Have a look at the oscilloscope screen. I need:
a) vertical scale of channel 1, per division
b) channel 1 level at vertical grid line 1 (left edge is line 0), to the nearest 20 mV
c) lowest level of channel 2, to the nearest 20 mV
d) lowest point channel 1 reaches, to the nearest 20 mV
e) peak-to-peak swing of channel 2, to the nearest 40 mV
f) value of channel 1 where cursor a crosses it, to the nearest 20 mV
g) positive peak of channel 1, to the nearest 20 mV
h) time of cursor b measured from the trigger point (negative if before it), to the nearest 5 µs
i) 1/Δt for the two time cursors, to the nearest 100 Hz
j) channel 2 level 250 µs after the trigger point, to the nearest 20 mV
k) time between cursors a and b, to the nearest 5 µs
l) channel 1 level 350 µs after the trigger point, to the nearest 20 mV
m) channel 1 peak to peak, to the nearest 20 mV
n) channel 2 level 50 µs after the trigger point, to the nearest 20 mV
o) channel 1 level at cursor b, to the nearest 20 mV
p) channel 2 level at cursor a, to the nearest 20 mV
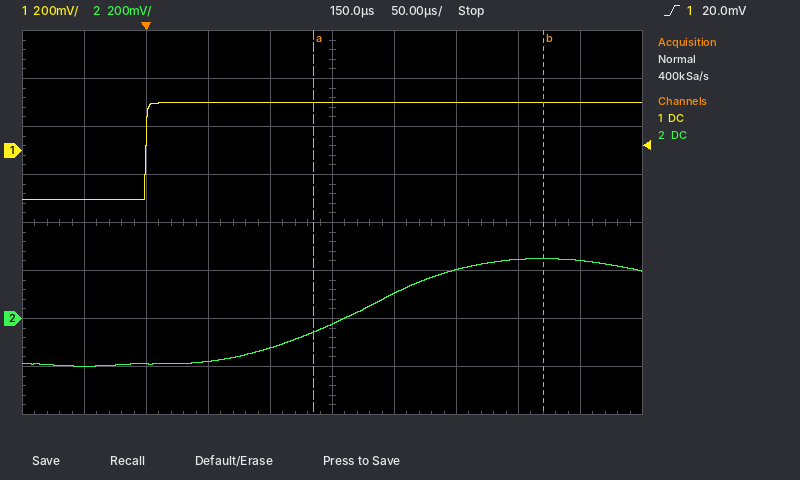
200 mV
-200 mV
-200 mV
-200 mV
440 mV
200 mV
200 mV
+320 µs
5.4 kHz
200 mV
185 µs
200 mV
400 mV
-180 mV
200 mV
-60 mV
